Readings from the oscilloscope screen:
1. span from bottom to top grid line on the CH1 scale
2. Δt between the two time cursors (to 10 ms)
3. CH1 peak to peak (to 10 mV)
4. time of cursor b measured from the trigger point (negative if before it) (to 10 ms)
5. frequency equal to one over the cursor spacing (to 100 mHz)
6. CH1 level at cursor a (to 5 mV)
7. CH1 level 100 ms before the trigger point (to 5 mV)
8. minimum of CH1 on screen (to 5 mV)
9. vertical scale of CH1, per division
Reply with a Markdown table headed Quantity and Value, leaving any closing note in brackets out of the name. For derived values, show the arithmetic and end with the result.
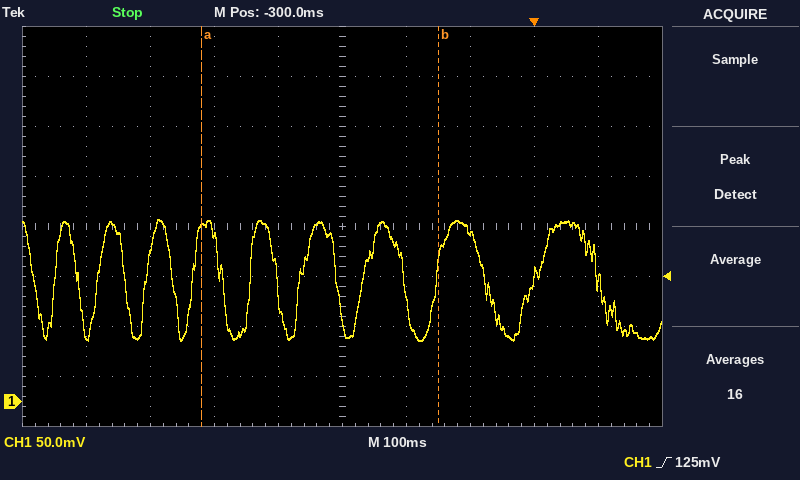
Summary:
| Quantity | Value |
|---|---|
| span from bottom to top grid line on the CH1 scale | 400 mV |
| Δt between the two time cursors | 370 ms |
| CH1 peak to peak | 120 mV |
| time of cursor b measured from the trigger point (negative if before it) | -150 ms |
| frequency equal to one over the cursor spacing | 1 / 370 ms ≈ 2.7 Hz |
| CH1 level at cursor a | 175 mV |
| CH1 level 100 ms before the trigger point | 170 mV |
| minimum of CH1 on screen | 60 mV |
| vertical scale of CH1, per division | 50 mV |
